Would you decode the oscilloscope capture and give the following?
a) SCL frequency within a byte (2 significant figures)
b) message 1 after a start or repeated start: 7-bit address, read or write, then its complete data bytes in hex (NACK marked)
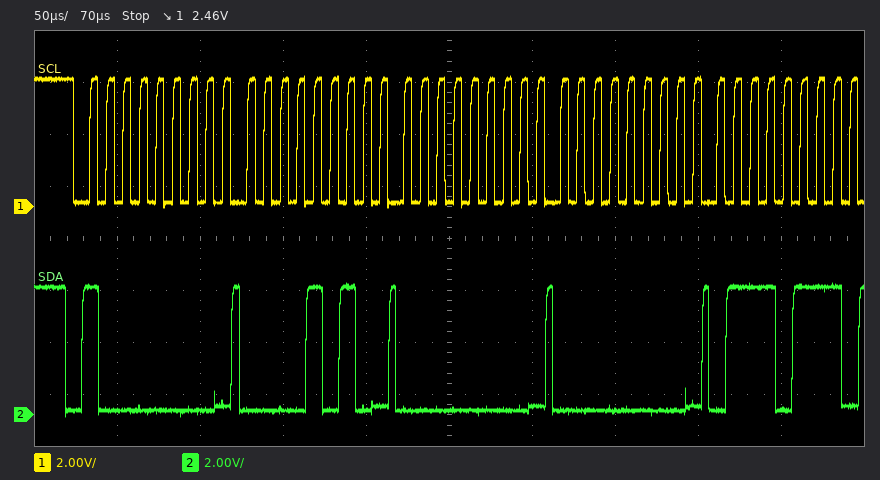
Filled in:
100 kHz
0x40 write: 0A 00 00 77
